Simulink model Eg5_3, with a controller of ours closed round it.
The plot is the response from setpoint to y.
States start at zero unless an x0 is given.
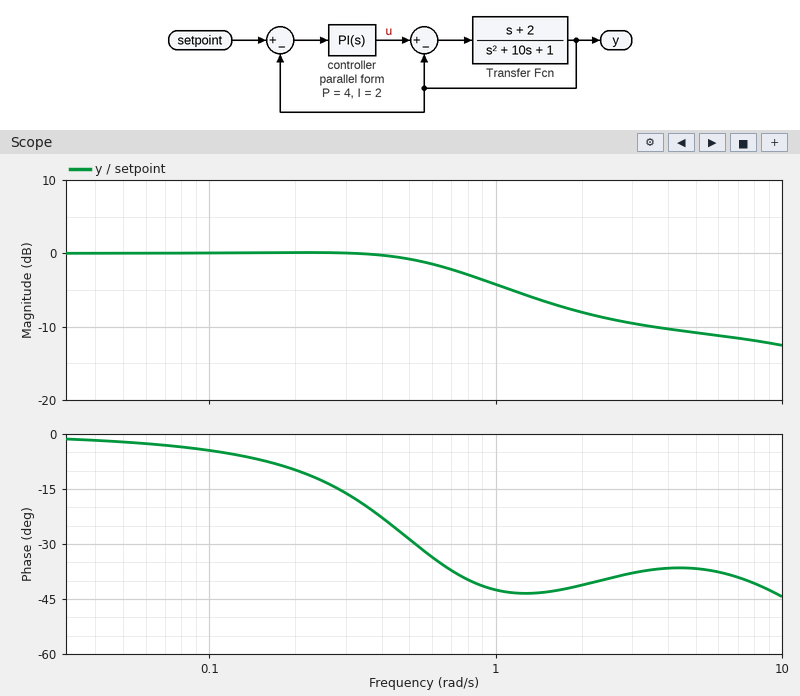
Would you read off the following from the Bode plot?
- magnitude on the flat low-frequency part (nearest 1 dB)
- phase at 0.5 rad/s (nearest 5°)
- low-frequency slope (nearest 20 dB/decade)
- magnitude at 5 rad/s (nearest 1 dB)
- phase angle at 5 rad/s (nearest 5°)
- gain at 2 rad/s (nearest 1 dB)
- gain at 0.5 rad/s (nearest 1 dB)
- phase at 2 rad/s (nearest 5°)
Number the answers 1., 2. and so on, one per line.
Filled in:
1. 0 dB
2. -30°
3. 0 dB/decade
4. -11 dB
5. -35°
6. -8 dB
7. -1 dB
8. -40°
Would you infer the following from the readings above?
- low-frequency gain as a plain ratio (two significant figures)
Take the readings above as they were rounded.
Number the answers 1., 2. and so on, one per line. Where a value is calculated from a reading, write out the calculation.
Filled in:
1. 10^(0 / 20) = 1.0
